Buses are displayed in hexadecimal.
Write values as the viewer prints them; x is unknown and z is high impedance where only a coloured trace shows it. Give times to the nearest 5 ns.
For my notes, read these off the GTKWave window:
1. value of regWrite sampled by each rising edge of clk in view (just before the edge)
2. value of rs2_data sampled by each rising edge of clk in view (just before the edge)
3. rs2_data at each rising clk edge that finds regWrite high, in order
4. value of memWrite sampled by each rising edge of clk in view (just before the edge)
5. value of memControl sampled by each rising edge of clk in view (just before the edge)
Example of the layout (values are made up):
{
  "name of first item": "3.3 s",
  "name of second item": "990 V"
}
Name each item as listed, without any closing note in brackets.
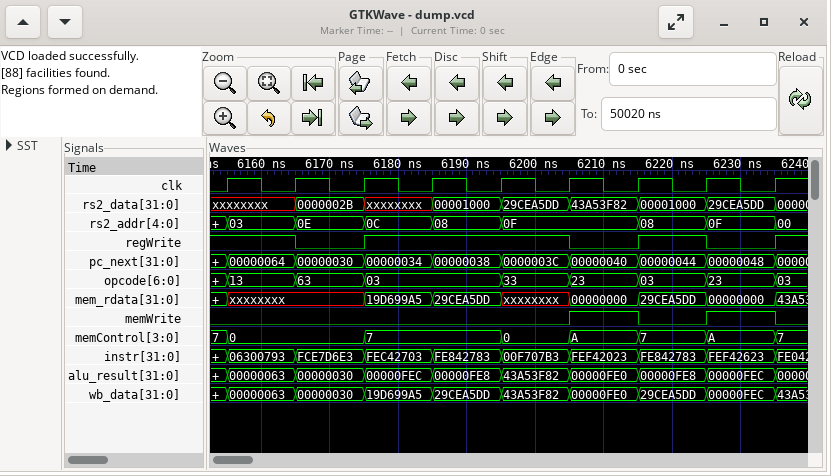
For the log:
{
  "value of regWrite sampled by each rising edge of clk in view": "1 1 0 1 1 1 0 1 0",
  "value of rs2_data sampled by each rising edge of clk in view": "xxxxxxxx, xxxxxxxx, 0000002B, xxxxxxxx, 00001000, 29CEA5DD, 43A53F82, 00001000, 29CEA5DD",
  "rs2_data at each rising clk edge that finds regWrite high, in order": "xxxxxxxx, xxxxxxxx, xxxxxxxx, 00001000, 29CEA5DD, 00001000",
  "value of memWrite sampled by each rising edge of clk in view": "0 0 0 0 0 0 1 0 1",
  "value of memControl sampled by each rising edge of clk in view": "7, 0, 0, 7, 7, 0, A, 7, A"
}
